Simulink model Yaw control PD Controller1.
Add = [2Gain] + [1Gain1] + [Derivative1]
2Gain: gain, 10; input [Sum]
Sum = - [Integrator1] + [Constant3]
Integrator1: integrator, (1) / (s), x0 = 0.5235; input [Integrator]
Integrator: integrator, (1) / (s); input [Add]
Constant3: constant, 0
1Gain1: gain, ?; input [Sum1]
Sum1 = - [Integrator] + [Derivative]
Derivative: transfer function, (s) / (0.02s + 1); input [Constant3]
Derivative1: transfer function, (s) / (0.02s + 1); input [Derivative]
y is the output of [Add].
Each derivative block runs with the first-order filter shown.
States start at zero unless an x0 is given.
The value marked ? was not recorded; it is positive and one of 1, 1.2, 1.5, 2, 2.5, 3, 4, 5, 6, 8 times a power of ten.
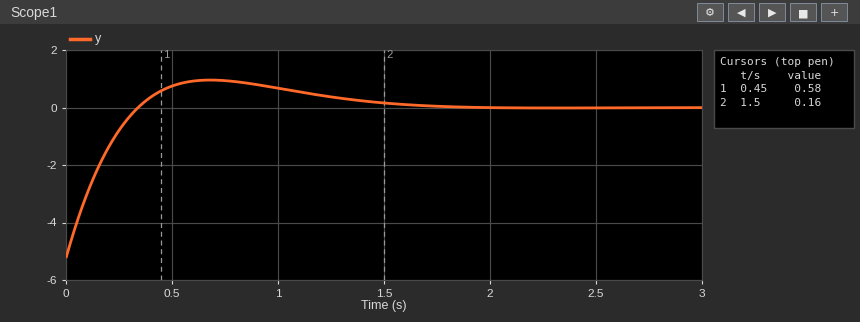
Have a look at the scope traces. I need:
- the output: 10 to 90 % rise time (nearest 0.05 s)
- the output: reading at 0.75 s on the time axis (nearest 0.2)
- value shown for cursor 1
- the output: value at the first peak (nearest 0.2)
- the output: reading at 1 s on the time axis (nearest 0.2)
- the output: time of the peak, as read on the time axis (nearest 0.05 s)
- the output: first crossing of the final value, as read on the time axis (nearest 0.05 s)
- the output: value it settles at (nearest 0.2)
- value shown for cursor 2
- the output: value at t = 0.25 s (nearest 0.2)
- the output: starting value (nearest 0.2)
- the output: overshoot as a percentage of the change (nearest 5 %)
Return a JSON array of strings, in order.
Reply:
["0.25 s", "1.0", "0.58", "1.0", "0.6", "0.70 s", "0.35 s", "0.0", "0.16", "-0.8", "-5.2", "20 %"]
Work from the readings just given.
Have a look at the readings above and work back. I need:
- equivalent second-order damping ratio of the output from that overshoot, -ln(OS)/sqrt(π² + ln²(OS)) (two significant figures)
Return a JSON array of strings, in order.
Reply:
["0.46"]
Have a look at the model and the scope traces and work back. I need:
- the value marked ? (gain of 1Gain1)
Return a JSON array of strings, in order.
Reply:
["5"]
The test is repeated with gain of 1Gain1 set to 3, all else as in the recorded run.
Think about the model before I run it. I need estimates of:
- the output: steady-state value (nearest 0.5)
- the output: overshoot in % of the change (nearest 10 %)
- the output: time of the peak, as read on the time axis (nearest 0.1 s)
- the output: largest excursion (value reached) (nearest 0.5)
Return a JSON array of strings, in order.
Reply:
["0.0", "30 %", "0.8 s", "1.5"]
